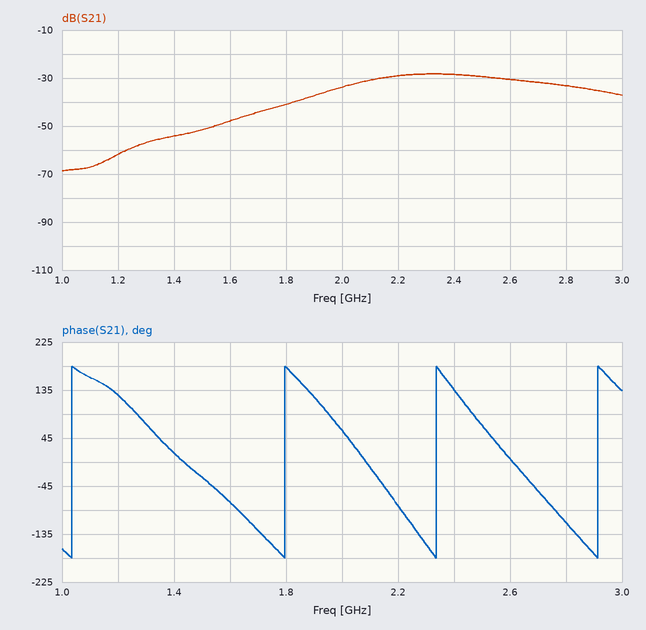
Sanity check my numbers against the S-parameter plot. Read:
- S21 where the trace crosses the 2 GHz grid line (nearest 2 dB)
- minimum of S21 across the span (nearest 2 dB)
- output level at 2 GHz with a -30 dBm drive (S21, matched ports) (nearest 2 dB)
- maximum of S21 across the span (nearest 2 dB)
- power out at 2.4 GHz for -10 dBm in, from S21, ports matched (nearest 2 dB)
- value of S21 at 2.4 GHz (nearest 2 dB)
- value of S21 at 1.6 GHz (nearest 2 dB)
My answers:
-34 dB
-68 dB
-64 dBm
-28 dB
-38 dBm
-28 dB
-48 dB
